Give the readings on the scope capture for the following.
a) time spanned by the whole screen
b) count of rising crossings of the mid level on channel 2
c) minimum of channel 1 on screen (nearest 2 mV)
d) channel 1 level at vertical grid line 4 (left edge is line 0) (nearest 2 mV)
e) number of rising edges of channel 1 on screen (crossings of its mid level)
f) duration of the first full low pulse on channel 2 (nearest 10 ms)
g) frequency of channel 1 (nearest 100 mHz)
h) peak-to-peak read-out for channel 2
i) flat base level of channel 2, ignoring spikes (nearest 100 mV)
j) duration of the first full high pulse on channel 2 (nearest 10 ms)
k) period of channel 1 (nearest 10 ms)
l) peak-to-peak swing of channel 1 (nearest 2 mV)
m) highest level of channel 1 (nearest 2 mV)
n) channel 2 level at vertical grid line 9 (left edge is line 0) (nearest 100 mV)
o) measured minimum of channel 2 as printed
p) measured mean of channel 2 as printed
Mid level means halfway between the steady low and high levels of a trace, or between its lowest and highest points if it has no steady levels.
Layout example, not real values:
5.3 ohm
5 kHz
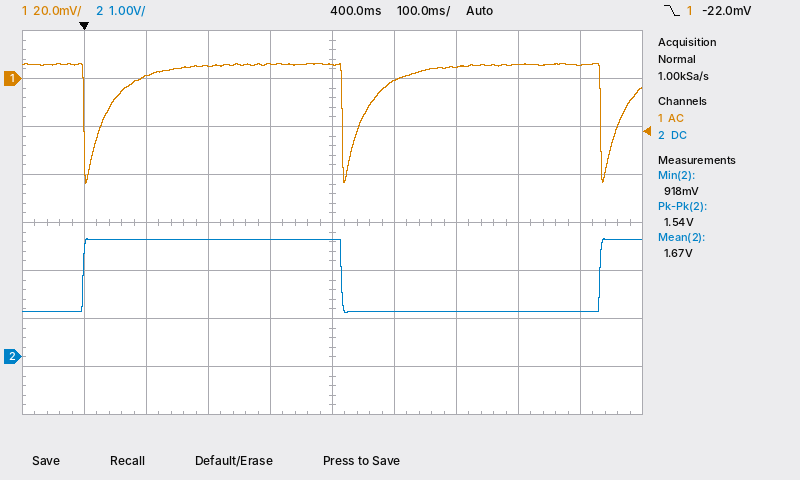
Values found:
1 s
2
-44 mV
6 mV
3
420 ms
2.4 Hz
1.54 V
900 mV
420 ms
420 ms
50 mV
6 mV
900 mV
918 mV
1.67 V
